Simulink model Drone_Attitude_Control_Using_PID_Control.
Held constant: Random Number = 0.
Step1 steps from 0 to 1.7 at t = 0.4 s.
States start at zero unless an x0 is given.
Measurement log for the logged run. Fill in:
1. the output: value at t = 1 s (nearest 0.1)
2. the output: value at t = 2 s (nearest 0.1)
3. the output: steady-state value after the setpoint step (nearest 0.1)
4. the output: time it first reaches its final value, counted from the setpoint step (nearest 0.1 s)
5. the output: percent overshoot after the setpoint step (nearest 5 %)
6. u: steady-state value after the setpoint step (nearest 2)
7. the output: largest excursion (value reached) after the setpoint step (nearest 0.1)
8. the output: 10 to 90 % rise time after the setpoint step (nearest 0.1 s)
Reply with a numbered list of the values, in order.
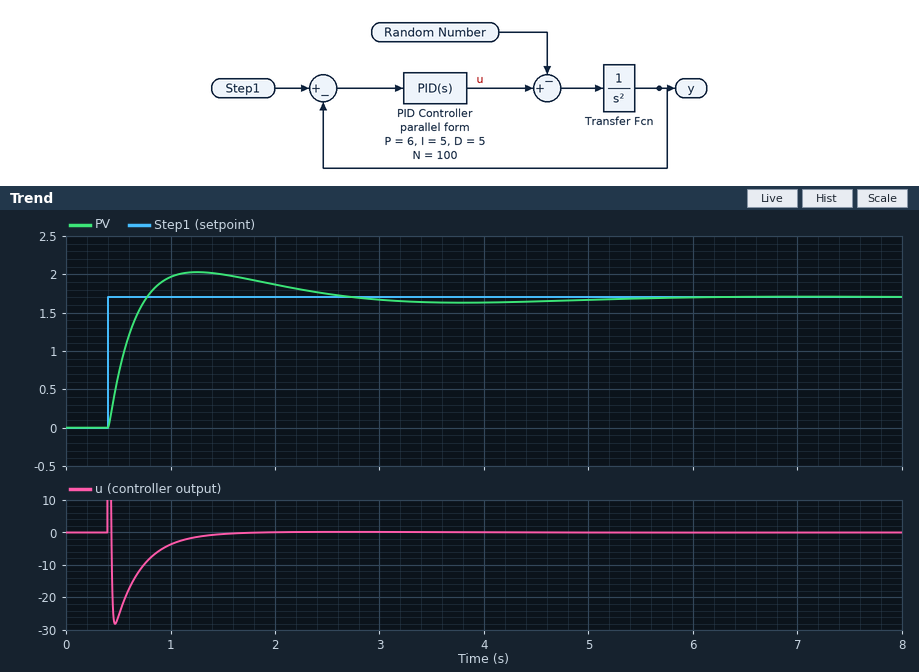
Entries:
1. 2.0
2. 1.9
3. 1.7
4. 0.4 s
5. 20 %
6. 0
7. 2.0
8. 0.3 s
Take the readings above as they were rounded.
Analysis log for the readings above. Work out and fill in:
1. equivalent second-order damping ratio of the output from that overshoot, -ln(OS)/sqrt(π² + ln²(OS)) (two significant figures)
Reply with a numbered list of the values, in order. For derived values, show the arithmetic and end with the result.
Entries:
1. ln(0.2) = -1.609; 1.609 / sqrt(9.870 + 2.590) = 0.46
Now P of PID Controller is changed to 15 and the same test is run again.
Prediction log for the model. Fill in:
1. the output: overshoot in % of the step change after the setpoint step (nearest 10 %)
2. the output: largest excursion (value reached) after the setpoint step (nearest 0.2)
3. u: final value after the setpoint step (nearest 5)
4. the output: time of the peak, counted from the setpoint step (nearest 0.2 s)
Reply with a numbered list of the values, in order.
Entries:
1. 30 %
2. 2.2
3. 0
4. 0.6 s
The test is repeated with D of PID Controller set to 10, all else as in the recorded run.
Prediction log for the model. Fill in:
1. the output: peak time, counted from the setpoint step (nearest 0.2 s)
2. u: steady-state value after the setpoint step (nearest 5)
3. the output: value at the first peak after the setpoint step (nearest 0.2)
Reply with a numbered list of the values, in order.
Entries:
1. 0.8 s
2. 0
3. 1.8
